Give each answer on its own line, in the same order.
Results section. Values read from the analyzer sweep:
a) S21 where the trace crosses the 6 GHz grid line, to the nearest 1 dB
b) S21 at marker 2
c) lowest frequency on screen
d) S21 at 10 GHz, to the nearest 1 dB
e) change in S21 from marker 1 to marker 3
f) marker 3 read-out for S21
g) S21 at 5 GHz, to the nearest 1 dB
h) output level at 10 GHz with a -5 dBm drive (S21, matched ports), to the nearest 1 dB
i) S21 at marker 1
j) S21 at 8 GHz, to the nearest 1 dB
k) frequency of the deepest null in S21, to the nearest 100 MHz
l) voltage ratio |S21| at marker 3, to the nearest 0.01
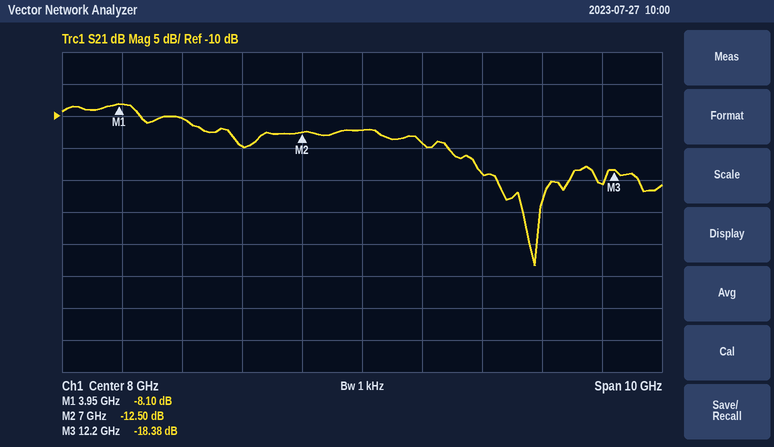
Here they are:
-15 dB
-12.50 dB
3 GHz
-19 dB
-10.28 dB
-18.38 dB
-10 dB
-24 dBm
-8.10 dB
-12 dB
10.9 GHz
0.12
